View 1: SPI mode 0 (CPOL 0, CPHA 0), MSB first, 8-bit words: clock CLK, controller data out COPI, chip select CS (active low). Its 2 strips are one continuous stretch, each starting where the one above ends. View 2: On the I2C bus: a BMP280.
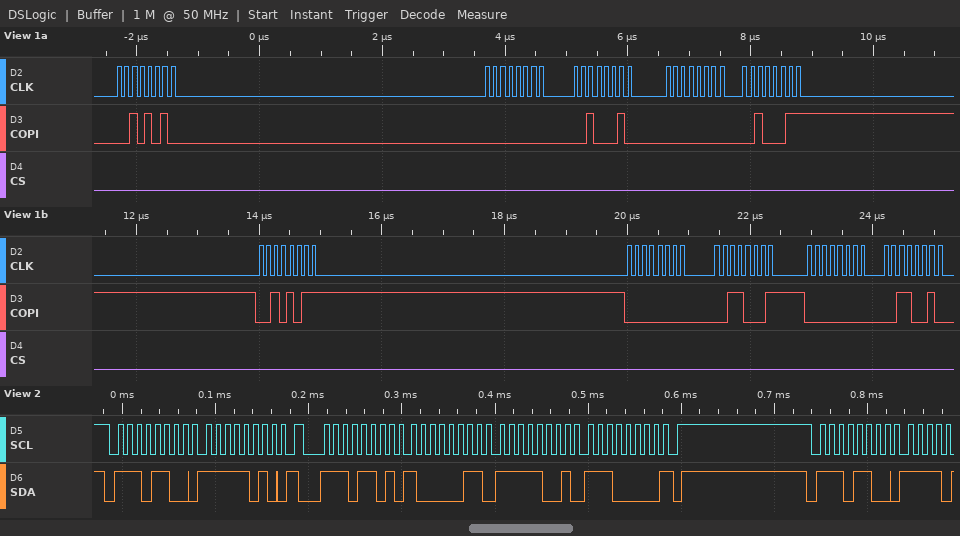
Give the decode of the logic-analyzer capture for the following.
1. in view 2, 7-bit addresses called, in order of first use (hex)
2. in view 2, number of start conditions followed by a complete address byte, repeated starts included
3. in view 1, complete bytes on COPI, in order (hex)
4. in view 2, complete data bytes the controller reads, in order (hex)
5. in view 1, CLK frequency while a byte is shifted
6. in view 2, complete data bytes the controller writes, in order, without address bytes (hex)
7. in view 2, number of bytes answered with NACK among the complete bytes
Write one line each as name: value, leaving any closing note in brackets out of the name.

in view 2, 7-bit addresses called, in order of first use: 0x76
in view 2, number of start conditions followed by a complete address byte, repeated starts included: 3
in view 1, complete bytes on COPI, in order: 0x2A 0x00 0x22 0x00 0x23 0x2B 0x00 0x31 0x00 0x32
in view 2, complete data bytes the controller reads, in order: 83 F9 E0
in view 1, CLK frequency while a byte is shifted: 8 MHz
in view 2, complete data bytes the controller writes, in order, without address bytes: FA
in view 2, number of bytes answered with NACK among the complete bytes: 1
